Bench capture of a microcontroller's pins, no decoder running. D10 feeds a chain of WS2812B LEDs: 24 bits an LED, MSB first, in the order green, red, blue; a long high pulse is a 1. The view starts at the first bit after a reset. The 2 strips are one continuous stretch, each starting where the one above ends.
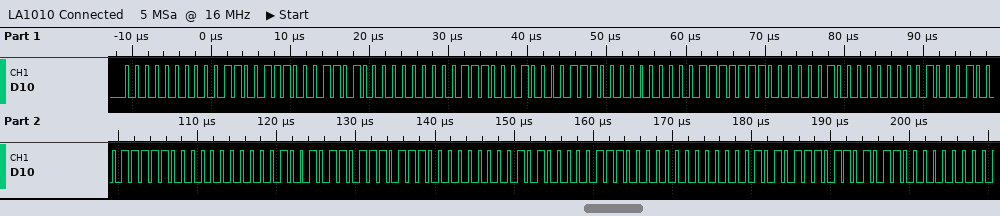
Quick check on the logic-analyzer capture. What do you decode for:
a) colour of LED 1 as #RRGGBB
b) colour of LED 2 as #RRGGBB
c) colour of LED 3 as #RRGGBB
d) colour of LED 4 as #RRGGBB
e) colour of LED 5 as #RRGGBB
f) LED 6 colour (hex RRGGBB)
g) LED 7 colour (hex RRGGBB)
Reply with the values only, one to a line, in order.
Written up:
#33008D
#380087
#3F0081
#44007C
#4B0077
#500070
#57006B
